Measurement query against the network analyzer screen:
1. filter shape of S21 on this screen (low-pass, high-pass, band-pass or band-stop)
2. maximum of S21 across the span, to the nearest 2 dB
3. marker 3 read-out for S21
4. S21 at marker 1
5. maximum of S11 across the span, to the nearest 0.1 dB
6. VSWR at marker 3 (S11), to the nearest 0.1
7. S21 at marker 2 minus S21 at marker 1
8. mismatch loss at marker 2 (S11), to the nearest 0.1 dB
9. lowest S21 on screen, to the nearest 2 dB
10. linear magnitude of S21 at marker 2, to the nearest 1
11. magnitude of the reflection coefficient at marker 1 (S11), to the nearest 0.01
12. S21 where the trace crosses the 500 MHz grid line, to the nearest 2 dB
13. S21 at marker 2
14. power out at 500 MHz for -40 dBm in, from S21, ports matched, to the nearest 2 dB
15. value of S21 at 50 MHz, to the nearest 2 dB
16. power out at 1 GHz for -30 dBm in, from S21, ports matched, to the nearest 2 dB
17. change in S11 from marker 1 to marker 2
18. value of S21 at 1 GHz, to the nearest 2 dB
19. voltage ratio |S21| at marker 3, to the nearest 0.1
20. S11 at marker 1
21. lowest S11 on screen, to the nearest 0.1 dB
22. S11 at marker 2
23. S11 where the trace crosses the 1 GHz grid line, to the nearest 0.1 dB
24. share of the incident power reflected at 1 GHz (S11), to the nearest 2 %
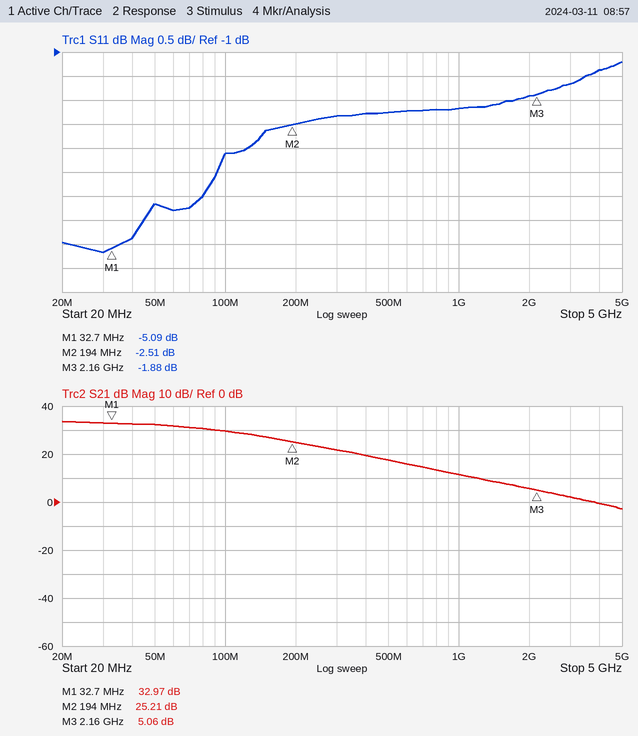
low-pass
34 dB
5.06 dB
32.97 dB
-1.2 dB
9.3
-7.76 dB
3.6 dB
-2 dB
18
0.56
18 dB
25.21 dB
-22 dBm
32 dB
-18 dBm
2.58 dB
12 dB
1.8
-5.09 dB
-5.2 dB
-2.51 dB
-2.2 dB
60 %
